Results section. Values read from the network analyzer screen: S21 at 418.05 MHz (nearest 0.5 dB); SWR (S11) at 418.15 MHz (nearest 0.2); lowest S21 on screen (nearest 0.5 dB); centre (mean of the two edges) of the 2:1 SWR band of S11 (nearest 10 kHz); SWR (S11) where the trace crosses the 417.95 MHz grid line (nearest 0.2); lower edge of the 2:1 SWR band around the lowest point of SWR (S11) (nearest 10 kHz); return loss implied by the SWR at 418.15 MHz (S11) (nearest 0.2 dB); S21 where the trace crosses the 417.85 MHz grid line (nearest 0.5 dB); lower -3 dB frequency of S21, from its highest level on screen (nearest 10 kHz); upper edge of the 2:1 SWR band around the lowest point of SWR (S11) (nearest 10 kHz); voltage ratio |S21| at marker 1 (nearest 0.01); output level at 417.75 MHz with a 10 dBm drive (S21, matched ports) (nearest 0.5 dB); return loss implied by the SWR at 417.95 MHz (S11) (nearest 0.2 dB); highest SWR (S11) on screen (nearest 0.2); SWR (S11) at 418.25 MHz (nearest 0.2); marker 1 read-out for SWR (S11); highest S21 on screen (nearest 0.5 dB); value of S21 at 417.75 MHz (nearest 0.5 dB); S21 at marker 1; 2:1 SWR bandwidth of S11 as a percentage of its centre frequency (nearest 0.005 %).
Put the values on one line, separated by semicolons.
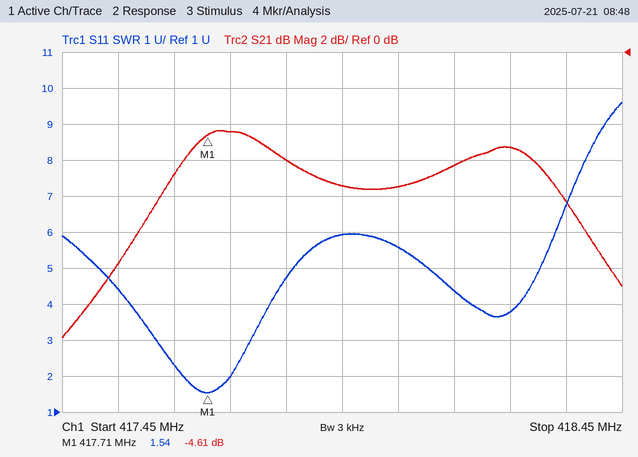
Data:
-7.5 dB; 4.4; -16.0 dB; 417.71 MHz; 6.0; 417.67 MHz; 4.0 dB; -6.0 dB; 417.64 MHz; 417.75 MHz; 0.59; 5.5 dBm; 3.0 dB; 9.6; 3.8; 1.54; -4.5 dB; -4.5 dB; -4.61 dB; 0.020 %
